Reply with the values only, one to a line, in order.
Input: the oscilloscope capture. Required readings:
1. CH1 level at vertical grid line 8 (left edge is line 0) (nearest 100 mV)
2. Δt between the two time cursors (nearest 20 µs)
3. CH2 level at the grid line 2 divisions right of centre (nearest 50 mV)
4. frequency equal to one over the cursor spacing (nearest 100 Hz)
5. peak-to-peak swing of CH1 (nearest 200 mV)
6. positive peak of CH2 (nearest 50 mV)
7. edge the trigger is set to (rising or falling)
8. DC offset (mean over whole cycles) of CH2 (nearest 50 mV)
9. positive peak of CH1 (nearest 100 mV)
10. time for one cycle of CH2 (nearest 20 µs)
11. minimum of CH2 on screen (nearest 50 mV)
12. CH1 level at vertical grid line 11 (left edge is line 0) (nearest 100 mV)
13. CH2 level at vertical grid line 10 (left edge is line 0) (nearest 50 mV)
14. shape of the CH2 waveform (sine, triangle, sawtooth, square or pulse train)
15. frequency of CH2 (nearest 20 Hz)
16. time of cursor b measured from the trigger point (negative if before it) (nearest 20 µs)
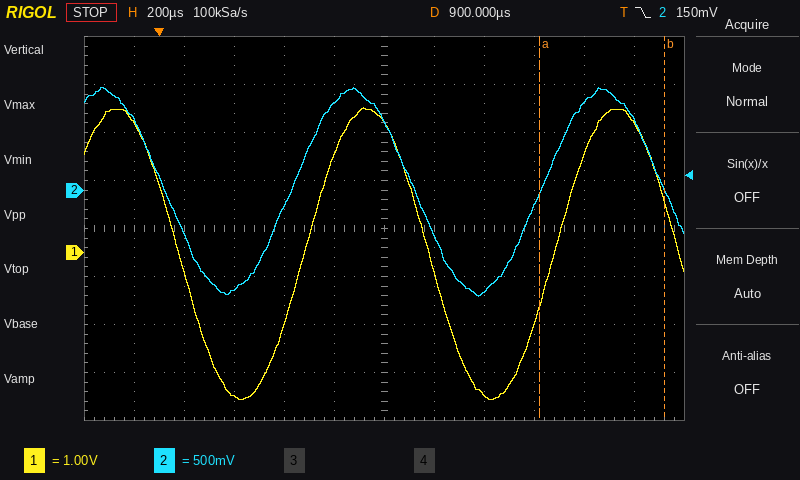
-3.0 V
500 µs
-1.05 V
2.0 kHz
6.0 V
1.05 V
falling
0 mV
3.0 V
1.00 ms
-1.10 V
2.7 V
900 mV
sine
1.00 kHz
+2.02 ms
